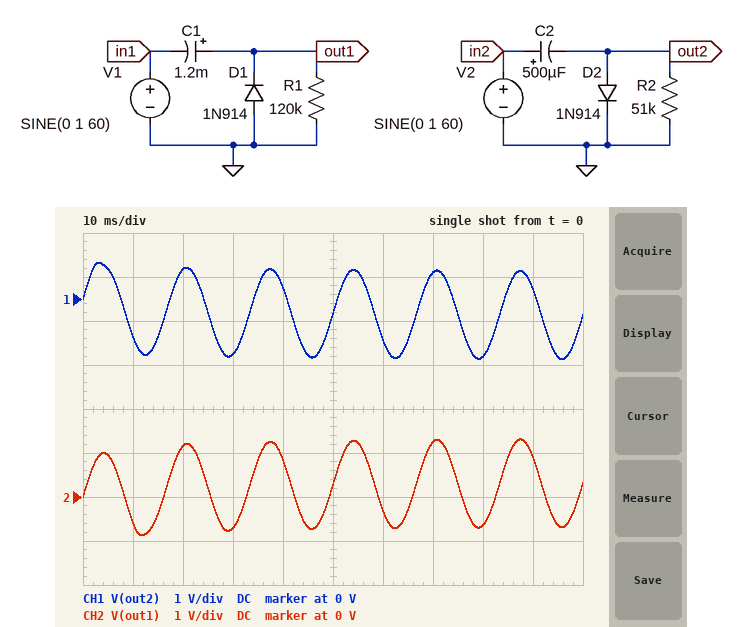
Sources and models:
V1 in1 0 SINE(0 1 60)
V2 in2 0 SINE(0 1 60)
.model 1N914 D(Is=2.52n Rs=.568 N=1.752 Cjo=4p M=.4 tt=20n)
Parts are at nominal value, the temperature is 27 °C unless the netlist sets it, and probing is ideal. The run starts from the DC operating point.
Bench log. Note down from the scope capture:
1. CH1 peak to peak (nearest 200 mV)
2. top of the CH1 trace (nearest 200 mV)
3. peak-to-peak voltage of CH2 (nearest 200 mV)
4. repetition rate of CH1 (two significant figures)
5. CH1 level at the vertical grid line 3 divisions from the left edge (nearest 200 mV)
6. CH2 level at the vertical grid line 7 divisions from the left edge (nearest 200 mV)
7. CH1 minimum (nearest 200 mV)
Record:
2.2 V
800 mV
2.2 V
60 Hz
-1.2 V
1.2 V
-1.4 V
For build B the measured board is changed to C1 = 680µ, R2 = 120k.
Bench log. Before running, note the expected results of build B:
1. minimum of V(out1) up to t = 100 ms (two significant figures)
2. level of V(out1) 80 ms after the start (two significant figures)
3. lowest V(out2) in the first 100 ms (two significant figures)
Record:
-840 mV
-610 mV
-1.4 V
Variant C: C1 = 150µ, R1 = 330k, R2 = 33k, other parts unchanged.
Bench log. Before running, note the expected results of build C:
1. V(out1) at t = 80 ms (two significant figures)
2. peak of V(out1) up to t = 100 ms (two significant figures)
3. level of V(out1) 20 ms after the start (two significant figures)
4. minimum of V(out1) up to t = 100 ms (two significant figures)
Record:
-540 mV
1.4 V
1.3 V
-750 mV
